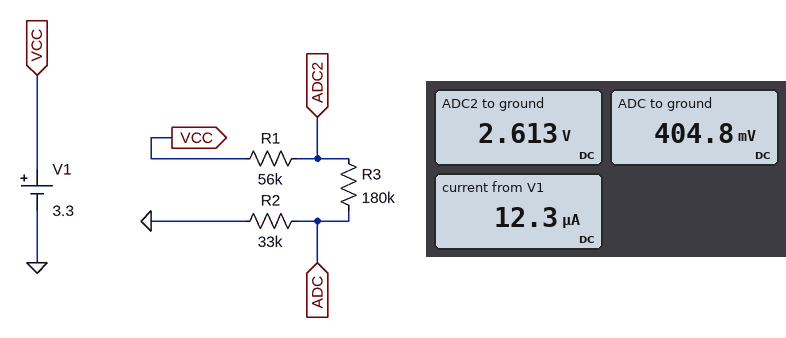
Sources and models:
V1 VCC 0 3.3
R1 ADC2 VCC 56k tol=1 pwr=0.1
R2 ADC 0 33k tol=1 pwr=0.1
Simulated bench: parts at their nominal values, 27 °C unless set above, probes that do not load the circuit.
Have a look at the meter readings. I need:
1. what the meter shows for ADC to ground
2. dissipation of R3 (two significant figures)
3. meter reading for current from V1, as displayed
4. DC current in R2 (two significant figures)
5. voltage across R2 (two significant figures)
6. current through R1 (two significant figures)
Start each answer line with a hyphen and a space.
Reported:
- 404.8 mV
- 27 µW
- 12.3 µA
- 12 µA
- 400 mV
- 12 µA
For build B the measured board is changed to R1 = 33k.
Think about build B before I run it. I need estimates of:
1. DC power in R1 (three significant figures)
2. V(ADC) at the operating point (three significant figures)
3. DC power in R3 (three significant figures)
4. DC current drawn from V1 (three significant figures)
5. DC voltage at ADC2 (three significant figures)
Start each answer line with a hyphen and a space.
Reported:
- 5.94 µW
- 443 mV
- 32.4 µW
- 13.4 µA
- 2.86 V
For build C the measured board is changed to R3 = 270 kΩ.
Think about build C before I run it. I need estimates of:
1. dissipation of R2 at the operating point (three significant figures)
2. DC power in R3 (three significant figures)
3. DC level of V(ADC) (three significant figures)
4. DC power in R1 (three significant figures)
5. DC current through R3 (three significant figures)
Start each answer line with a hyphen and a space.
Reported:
- 2.79 µW
- 22.8 µW
- 303 mV
- 4.73 µW
- 9.19 µA
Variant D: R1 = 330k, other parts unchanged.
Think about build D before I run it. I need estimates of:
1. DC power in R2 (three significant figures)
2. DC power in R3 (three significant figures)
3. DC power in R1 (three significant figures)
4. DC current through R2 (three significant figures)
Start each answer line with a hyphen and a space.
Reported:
- 1.22 µW
- 6.65 µW
- 12.2 µW
- 6.08 µA
